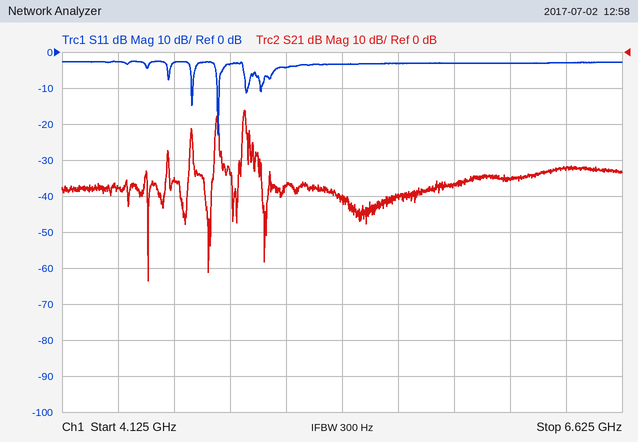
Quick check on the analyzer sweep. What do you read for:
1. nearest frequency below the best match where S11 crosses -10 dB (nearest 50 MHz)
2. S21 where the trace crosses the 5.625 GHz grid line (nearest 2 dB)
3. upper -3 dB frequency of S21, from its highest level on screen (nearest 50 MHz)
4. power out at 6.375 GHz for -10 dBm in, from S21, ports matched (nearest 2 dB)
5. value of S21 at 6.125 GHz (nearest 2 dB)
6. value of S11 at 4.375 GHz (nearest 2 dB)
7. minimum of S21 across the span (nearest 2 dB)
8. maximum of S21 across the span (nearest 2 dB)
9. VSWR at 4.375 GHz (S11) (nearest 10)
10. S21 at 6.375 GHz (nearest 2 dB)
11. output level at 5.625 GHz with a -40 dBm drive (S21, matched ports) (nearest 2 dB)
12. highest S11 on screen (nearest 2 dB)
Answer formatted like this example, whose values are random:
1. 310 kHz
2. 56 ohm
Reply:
1. 4.80 GHz
2. -40 dB
3. 4.95 GHz
4. -42 dBm
5. -36 dB
6. -2 dB
7. -64 dB
8. -16 dB
9. 10
10. -32 dB
11. -80 dBm
12. -2 dB
